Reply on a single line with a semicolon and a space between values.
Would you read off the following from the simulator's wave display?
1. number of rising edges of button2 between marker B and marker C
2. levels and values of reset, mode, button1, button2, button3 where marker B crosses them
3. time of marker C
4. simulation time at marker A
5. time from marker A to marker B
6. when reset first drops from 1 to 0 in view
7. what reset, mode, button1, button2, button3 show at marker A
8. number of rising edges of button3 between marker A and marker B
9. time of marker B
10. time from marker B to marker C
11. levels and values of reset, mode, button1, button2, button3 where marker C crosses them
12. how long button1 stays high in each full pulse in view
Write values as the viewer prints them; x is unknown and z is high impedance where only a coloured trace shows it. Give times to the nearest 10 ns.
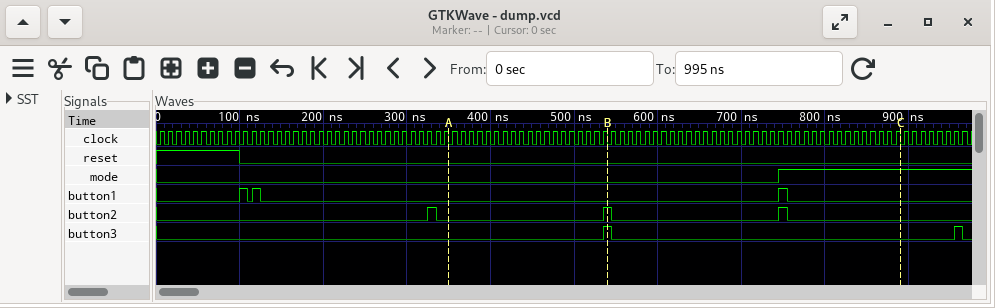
1; reset=0, mode=0, button1=0, button2=1, button3=1; 890 ns; 350 ns; 190 ns; 100 ns; reset=0, mode=0, button1=0, button2=0, button3=0; 1; 540 ns; 350 ns; reset=0, mode=1, button1=0, button2=0, button3=0; 10 ns, 10 ns, 10 ns
